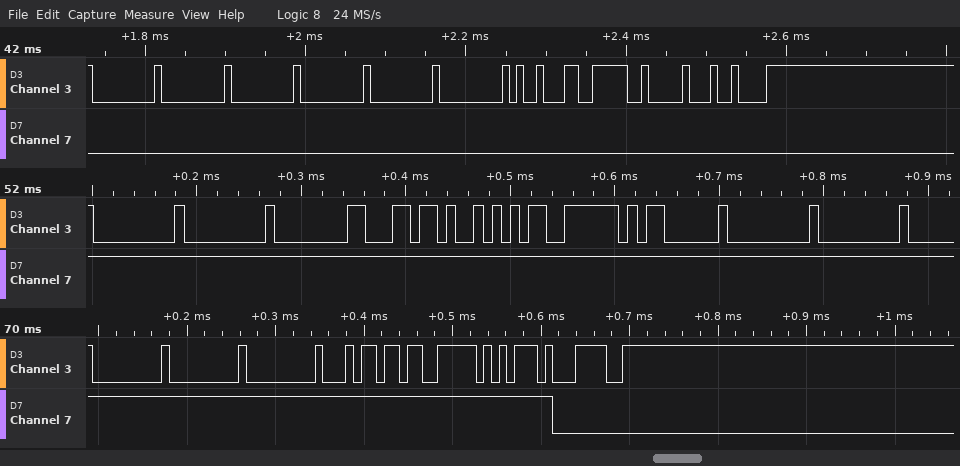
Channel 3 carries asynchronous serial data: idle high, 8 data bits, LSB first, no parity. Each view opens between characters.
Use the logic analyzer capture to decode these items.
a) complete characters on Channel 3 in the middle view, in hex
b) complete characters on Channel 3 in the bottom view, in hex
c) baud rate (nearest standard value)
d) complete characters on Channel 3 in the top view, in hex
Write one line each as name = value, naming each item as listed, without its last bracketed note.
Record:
complete characters on Channel 3 in the middle view, in hex = 00, 00, 80, 6C, AA, 7E, 03, 00, 00
complete characters on Channel 3 in the bottom view, in hex = 00, 00, 00, B4, F3, 75, 3C
baud rate = 115200 baud
complete characters on Channel 3 in the top view, in hex = 00, 00, 00, 00, 00, 00, 89, 3E, 10, C2
